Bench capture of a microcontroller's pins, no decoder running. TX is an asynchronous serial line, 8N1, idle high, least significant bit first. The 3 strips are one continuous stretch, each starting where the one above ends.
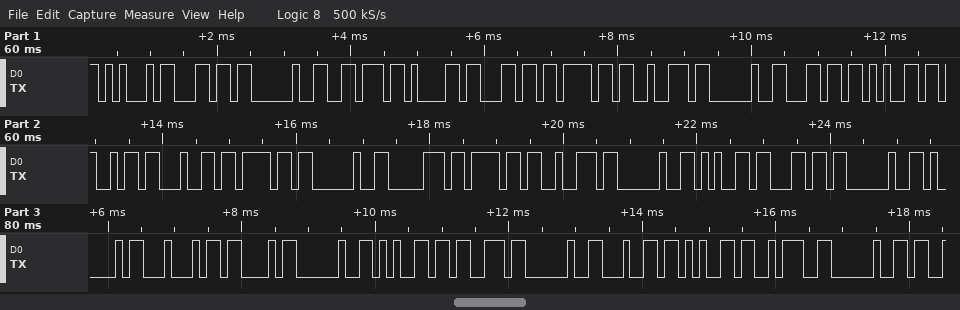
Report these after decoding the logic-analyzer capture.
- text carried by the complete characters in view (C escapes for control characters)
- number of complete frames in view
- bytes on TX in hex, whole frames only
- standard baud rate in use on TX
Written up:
"El valor leido por el ADC es de: "
33
45 6C 20 76 61 6C 6F 72 20 6C 65 69 64 6F 20 70 6F 72 20 65 6C 20 41 44 43 20 65 73 20 64 65 3A 20
9600 baud
